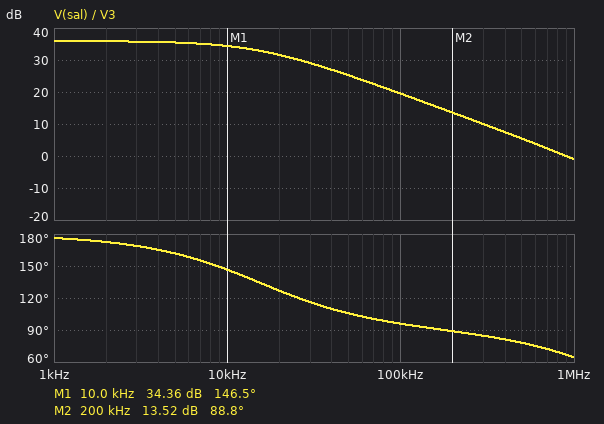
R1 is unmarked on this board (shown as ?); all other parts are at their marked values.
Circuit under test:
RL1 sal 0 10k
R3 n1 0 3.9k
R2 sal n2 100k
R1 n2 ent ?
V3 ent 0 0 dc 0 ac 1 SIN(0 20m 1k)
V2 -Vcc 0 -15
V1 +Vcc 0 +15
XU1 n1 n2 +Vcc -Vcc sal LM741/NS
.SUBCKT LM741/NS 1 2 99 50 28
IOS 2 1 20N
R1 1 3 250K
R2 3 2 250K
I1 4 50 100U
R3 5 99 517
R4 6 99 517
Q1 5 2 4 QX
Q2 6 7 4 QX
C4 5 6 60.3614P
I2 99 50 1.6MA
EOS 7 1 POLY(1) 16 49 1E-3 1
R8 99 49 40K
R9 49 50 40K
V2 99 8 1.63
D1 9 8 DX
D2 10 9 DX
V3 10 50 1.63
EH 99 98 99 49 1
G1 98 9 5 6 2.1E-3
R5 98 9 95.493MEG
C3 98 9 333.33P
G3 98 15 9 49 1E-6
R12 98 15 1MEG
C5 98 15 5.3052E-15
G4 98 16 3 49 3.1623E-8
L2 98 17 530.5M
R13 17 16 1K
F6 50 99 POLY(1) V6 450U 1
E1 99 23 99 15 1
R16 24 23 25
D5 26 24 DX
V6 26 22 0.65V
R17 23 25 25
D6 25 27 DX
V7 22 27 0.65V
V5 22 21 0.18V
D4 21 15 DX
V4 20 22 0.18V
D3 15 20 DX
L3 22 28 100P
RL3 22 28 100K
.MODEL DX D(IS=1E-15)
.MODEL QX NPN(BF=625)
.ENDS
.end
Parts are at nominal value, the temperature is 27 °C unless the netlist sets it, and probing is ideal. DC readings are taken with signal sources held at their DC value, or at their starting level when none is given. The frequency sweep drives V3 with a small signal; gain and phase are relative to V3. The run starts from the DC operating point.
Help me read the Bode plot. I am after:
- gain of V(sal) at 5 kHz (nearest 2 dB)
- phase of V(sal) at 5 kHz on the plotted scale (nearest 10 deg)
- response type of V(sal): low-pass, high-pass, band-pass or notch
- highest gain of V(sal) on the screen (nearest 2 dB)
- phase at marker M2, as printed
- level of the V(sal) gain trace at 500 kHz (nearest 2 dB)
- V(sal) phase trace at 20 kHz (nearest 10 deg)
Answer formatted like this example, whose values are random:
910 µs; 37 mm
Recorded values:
36 dB; 160 deg; low-pass; 36 dB; 88.8 deg; 6 dB; 130 deg
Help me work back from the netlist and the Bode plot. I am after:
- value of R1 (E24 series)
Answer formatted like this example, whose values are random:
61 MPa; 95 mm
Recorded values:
1.6 kΩ
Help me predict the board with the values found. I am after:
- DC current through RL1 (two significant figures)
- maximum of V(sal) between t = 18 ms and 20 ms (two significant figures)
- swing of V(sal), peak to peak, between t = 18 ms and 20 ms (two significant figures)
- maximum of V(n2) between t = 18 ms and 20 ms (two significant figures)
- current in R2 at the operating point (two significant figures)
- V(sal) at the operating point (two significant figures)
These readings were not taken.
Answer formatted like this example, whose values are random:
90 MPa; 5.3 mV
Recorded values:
5.9 µA; 1.3 V; 2.5 V; 2.1 mV; 590 nA; 59 mV
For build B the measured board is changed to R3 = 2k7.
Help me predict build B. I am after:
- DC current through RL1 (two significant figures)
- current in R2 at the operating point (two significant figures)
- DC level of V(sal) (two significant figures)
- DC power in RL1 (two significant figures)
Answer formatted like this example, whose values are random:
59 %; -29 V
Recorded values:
6.4 µA; 630 nA; 64 mV; 410 nW
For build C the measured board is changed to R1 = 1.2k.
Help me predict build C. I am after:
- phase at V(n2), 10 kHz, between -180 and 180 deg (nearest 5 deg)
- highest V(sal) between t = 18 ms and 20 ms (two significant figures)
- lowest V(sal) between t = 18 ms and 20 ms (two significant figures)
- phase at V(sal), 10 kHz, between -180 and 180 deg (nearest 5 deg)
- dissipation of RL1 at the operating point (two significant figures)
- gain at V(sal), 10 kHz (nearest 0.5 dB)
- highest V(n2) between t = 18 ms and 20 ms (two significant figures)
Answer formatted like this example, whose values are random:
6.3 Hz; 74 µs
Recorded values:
50 deg; 1.7 V; -1.6 V; 140 deg; 570 nW; 36.0 dB; 2.5 mV
